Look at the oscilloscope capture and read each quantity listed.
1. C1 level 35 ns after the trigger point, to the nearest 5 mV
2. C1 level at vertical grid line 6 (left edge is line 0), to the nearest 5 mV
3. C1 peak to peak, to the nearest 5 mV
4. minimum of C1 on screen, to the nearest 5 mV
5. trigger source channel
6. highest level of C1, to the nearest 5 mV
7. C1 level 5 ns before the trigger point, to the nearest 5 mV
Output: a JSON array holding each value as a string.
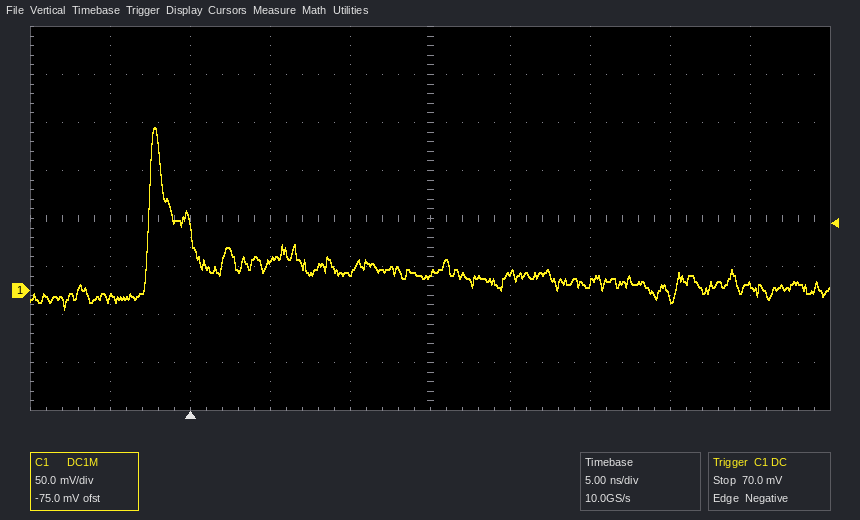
["5 mV", "20 mV", "190 mV", "-20 mV", "C1", "170 mV", "-10 mV"]
